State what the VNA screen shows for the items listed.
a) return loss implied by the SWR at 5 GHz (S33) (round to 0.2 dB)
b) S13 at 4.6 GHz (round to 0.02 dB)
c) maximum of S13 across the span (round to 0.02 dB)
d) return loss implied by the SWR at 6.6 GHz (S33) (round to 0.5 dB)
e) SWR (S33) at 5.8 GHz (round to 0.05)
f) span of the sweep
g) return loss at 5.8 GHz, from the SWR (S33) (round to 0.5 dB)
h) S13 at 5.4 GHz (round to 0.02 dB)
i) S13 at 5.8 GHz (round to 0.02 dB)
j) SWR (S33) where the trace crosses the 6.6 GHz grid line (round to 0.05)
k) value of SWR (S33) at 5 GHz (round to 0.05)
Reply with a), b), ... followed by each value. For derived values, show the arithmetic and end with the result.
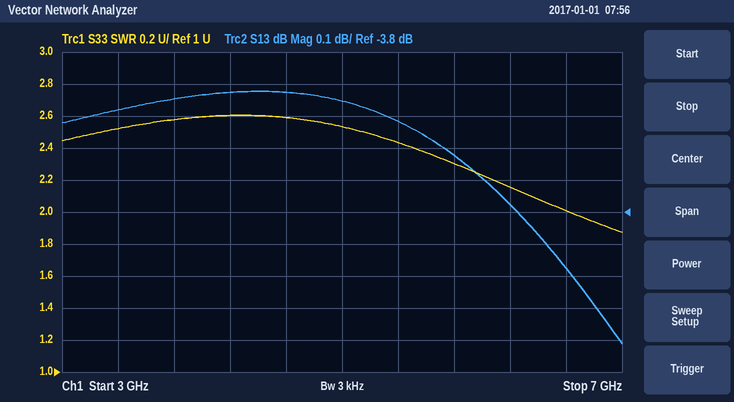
a) −20 log10((2.55 − 1)/(2.55 + 1)) ≈ 7.2 dB
b) -3.42 dB
c) -3.42 dB
d) −20 log10((2 − 1)/(2 + 1)) ≈ 9.5 dB
e) 2.30
f) 4 GHz
g) −20 log10((2.3 − 1)/(2.3 + 1)) ≈ 8.09 dB, so 8.0 dB to the nearest 0.5 dB
h) -3.52 dB
i) -3.62 dB
j) 2.00
k) 2.55
